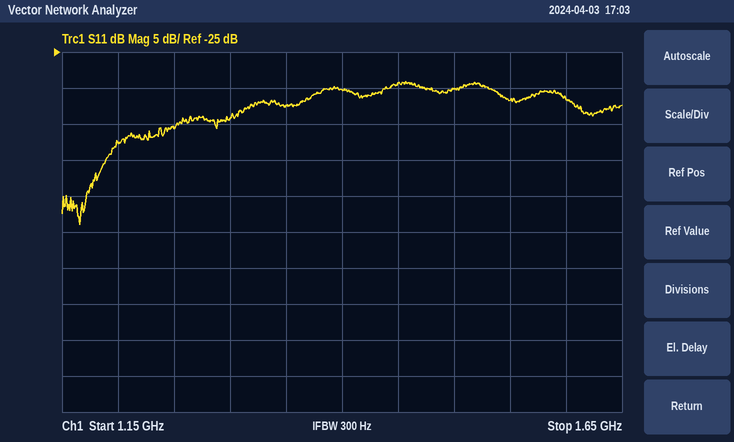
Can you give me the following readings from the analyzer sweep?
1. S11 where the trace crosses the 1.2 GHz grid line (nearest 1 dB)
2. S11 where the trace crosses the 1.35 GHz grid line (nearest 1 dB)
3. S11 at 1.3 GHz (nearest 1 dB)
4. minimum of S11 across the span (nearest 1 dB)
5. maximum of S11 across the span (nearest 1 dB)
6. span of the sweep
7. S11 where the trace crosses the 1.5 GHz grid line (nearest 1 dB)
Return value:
-38 dB
-32 dB
-34 dB
-49 dB
-29 dB
500 MHz
-30 dB
